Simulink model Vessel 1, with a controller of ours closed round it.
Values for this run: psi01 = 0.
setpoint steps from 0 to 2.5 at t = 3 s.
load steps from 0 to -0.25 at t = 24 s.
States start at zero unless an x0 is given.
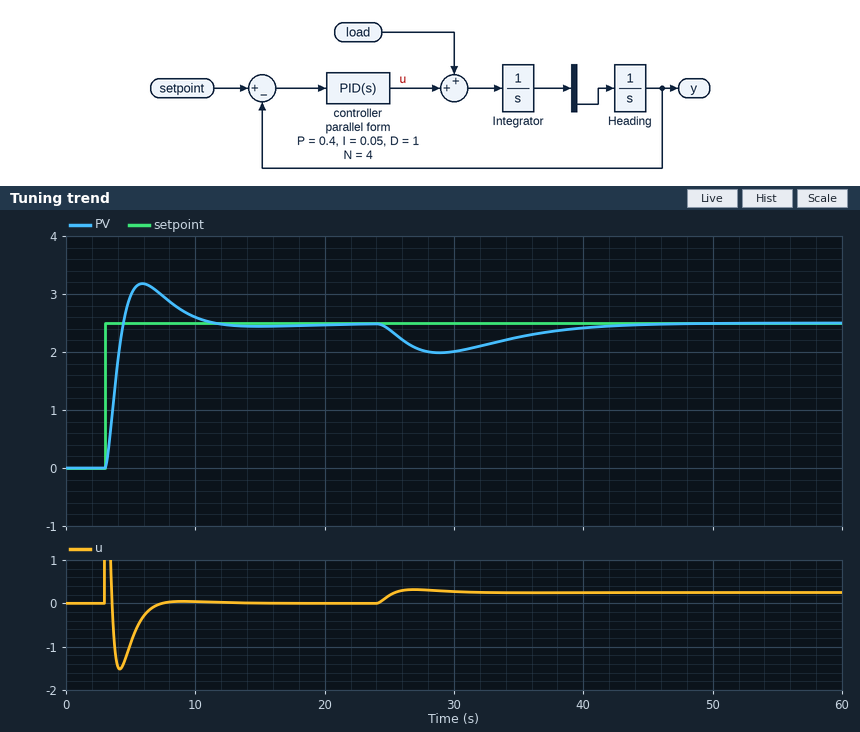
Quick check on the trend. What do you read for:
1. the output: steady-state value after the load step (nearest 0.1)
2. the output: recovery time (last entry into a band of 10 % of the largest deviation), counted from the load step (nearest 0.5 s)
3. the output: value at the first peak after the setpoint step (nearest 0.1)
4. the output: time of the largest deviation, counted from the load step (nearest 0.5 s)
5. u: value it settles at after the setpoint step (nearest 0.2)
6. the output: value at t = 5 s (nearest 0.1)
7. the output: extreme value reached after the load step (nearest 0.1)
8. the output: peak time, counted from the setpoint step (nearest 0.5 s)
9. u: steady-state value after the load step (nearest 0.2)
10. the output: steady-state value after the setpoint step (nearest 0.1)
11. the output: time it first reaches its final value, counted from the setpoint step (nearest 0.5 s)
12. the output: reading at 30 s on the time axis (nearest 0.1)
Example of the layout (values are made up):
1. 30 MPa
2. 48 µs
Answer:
1. 2.5
2. 18.5 s
3. 3.2
4. 5.0 s
5. 0.0
6. 3.0
7. 2.0
8. 3.0 s
9. 0.2
10. 2.5
11. 1.5 s
12. 2.0
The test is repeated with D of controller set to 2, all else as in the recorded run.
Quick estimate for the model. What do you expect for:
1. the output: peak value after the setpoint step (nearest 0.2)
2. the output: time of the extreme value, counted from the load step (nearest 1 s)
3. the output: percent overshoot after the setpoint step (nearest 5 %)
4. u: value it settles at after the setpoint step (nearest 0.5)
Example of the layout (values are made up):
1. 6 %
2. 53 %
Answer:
1. 2.8
2. 7 s
3. 15 %
4. 0.0
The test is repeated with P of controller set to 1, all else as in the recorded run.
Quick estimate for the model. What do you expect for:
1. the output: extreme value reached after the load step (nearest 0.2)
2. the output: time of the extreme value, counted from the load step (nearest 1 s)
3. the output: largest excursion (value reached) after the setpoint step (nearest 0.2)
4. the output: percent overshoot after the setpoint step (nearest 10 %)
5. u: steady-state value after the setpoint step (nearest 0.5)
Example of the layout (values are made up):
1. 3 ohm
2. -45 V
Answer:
1. 2.2
2. 3 s
3. 3.6
4. 40 %
5. 0.0
